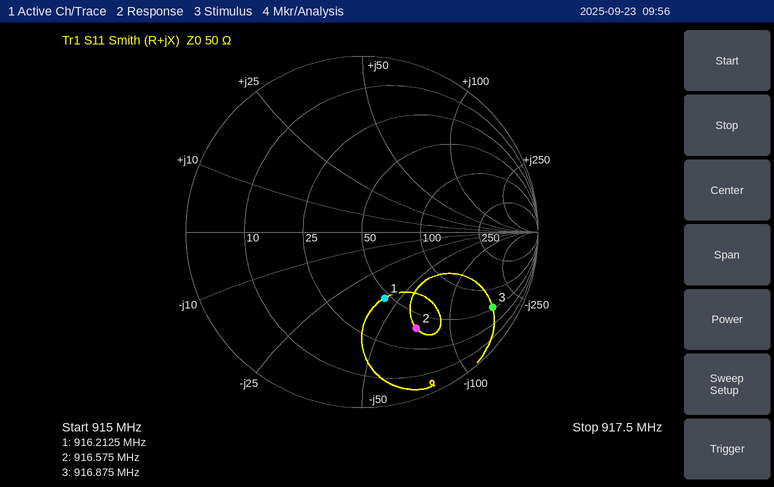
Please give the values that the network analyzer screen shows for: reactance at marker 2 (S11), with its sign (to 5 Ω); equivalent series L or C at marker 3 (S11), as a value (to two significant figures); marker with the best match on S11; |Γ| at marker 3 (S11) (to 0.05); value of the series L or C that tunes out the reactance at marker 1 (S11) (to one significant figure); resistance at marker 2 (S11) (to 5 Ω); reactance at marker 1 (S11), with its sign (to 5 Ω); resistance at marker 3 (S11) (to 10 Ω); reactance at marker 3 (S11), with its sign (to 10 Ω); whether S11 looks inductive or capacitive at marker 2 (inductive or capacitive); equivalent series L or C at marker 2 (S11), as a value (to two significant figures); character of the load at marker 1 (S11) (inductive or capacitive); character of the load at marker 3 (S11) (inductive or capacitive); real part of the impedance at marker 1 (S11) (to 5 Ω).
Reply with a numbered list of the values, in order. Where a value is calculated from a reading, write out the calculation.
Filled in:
1. -70 Ω
2. C = 1/(2π × 916.875 MHz × 170 Ω) ≈ 1.0 pF
3. marker 1
4. 0.85
5. L = 40 Ω/(2π × 916.2125 MHz) ≈ 7 nH
6. 40 Ω
7. -40 Ω
8. 50 Ω
9. -170 Ω
10. capacitive
11. C = 1/(2π × 916.575 MHz × 70 Ω) ≈ 2.5 pF
12. capacitive
13. capacitive
14. 45 Ω
